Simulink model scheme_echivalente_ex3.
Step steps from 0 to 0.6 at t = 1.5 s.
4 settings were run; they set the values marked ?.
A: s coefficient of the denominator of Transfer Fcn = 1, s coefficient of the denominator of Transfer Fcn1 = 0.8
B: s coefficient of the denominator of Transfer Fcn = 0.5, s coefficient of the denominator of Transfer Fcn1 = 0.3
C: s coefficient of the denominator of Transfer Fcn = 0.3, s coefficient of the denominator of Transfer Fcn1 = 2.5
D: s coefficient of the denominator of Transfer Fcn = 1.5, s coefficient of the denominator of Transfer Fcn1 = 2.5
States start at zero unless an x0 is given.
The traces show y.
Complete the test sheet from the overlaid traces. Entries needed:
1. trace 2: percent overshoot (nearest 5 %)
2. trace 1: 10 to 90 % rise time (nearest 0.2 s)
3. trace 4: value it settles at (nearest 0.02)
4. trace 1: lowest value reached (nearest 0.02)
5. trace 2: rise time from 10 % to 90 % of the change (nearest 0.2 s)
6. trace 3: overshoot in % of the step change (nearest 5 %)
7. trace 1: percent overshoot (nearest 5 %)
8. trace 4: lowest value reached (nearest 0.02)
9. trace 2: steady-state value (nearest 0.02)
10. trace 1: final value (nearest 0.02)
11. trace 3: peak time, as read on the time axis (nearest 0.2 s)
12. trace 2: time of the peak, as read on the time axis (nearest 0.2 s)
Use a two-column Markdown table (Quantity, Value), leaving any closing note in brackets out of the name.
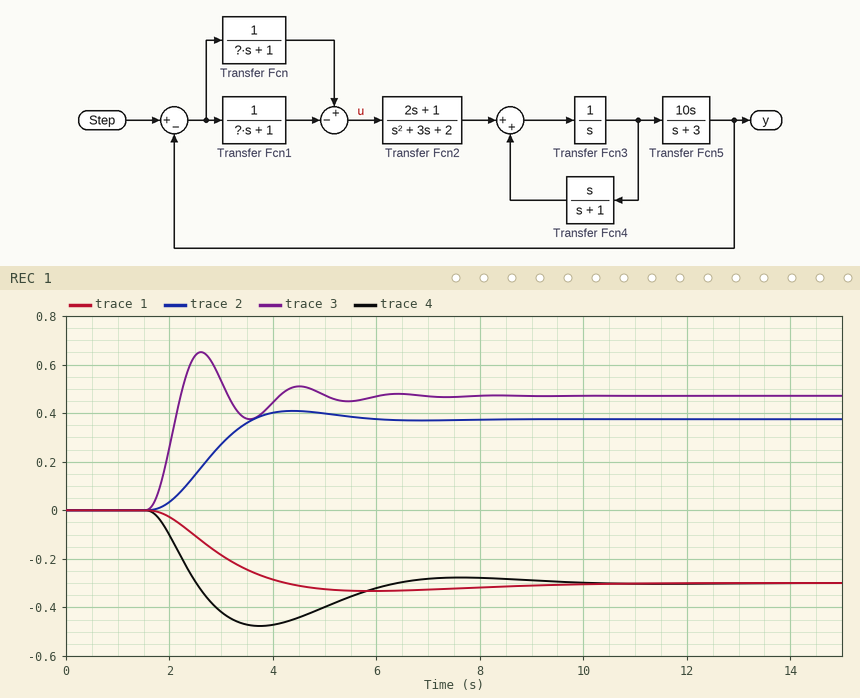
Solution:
| Quantity | Value |
|---|---|
| trace 2: percent overshoot | 10 % |
| trace 1: 10 to 90 % rise time | 1.8 s |
| trace 4: value it settles at | -0.30 |
| trace 1: lowest value reached | -0.34 |
| trace 2: rise time from 10 % to 90 % of the change | 1.4 s |
| trace 3: overshoot in % of the step change | 40 % |
| trace 1: percent overshoot | 10 % |
| trace 4: lowest value reached | -0.48 |
| trace 2: steady-state value | 0.38 |
| trace 1: final value | -0.30 |
| trace 3: peak time, as read on the time axis | 2.6 s |
| trace 2: time of the peak, as read on the time axis | 4.4 s |
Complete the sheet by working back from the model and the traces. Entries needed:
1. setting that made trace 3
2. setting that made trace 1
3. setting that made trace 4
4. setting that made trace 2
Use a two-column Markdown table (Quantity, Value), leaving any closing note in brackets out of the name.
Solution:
| Quantity | Value |
|---|---|
| setting that made trace 3 | C |
| setting that made trace 1 | A |
| setting that made trace 4 | B |
| setting that made trace 2 | D |
